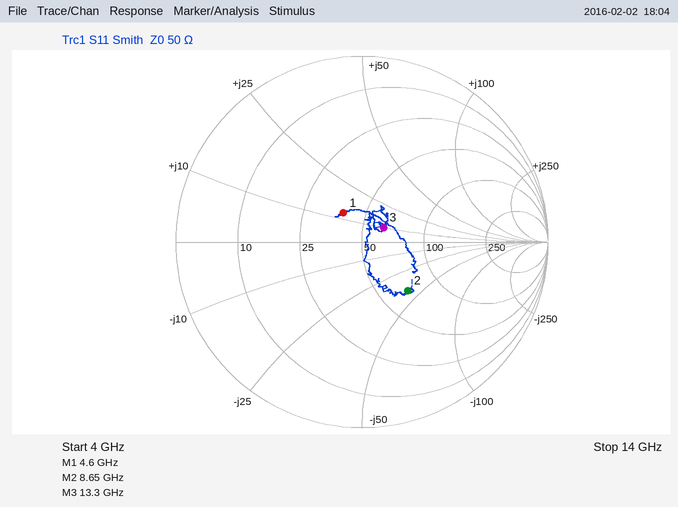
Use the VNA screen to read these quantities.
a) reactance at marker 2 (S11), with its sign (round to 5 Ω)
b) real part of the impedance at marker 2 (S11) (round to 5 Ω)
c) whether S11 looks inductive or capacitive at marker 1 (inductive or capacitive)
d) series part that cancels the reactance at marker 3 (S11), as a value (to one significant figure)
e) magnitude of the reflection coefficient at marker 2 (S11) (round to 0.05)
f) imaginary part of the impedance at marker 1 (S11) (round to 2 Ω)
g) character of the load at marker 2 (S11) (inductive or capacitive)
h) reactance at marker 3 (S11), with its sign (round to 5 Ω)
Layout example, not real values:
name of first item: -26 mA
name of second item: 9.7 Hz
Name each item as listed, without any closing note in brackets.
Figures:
reactance at marker 2 (S11), with its sign: -40 Ω
real part of the impedance at marker 2 (S11): 70 Ω
whether S11 looks inductive or capacitive at marker 1: inductive
series part that cancels the reactance at marker 3 (S11), as a value: 1 pF
magnitude of the reflection coefficient at marker 2 (S11): 0.35
imaginary part of the impedance at marker 1 (S11): +12 Ω
character of the load at marker 2 (S11): capacitive
reactance at marker 3 (S11), with its sign: +10 Ω
